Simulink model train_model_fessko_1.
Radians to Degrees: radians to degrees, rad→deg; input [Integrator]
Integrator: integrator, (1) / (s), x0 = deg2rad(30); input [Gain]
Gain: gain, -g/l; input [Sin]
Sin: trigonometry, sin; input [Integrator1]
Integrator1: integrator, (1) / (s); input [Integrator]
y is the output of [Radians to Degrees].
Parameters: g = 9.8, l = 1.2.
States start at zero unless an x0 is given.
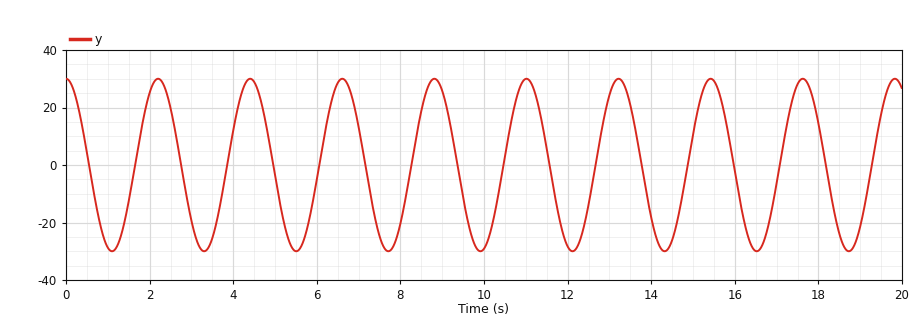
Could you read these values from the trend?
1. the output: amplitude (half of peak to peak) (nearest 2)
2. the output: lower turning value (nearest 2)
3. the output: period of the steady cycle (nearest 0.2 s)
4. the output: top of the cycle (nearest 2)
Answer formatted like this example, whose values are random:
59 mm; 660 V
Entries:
30; -30; 2.2 s; 30
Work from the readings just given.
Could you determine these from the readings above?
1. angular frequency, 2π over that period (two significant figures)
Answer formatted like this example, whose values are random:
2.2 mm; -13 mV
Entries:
2.9 rad/s
